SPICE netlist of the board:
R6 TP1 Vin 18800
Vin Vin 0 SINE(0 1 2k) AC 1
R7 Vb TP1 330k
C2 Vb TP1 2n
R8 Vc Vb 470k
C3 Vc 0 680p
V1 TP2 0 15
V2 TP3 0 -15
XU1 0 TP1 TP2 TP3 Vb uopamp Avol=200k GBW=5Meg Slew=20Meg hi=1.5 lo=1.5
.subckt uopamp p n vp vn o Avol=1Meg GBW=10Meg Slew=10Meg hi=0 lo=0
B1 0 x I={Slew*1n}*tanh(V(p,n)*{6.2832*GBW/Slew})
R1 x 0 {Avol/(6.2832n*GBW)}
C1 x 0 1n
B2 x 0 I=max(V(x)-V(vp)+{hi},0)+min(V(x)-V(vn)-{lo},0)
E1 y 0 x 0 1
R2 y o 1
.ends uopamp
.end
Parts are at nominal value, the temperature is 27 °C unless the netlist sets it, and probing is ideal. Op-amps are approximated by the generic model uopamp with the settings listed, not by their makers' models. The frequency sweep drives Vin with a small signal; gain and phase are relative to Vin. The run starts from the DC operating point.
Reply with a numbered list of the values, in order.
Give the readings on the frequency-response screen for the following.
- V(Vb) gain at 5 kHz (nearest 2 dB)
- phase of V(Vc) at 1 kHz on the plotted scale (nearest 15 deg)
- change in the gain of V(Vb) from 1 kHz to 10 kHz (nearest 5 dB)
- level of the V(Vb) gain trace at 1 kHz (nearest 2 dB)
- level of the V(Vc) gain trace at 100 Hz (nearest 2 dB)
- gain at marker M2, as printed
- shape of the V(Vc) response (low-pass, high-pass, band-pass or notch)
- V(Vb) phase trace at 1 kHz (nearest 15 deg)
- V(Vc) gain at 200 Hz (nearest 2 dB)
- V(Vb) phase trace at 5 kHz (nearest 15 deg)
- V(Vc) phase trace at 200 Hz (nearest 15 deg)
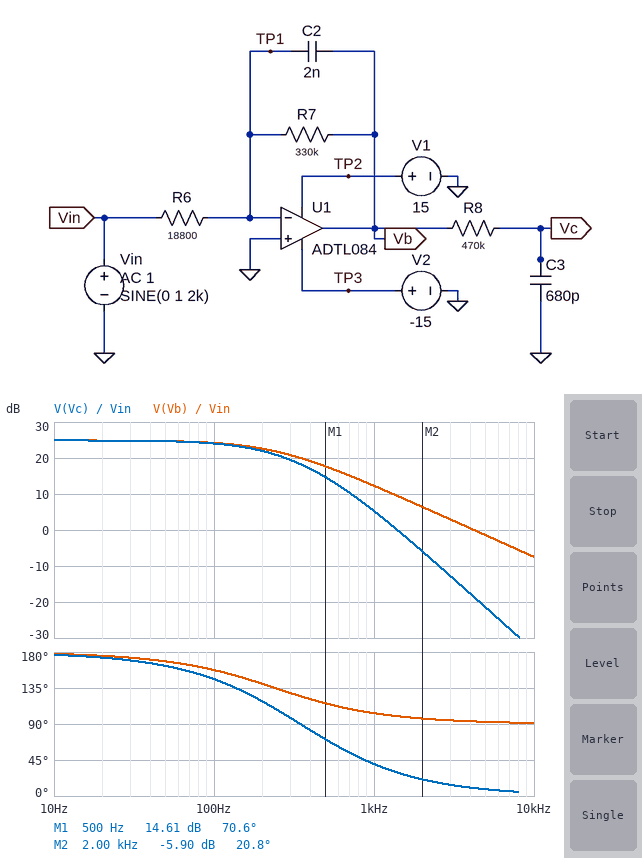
1. -2 dB
2. 45 deg
3. -20 dB
4. 12 dB
5. 24 dB
6. -5.90 dB
7. low-pass
8. 105 deg
9. 22 dB
10. 90 deg
11. 120 deg
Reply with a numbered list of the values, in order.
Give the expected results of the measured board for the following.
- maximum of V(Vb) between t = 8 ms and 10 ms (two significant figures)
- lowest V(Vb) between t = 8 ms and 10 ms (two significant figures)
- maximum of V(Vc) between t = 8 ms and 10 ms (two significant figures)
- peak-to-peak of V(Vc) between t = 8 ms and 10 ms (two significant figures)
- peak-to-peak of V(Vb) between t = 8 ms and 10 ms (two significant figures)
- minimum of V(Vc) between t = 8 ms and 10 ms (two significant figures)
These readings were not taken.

1. 2.1 V
2. -2.1 V
3. 510 mV
4. 1.0 V
5. 4.2 V
6. -510 mV
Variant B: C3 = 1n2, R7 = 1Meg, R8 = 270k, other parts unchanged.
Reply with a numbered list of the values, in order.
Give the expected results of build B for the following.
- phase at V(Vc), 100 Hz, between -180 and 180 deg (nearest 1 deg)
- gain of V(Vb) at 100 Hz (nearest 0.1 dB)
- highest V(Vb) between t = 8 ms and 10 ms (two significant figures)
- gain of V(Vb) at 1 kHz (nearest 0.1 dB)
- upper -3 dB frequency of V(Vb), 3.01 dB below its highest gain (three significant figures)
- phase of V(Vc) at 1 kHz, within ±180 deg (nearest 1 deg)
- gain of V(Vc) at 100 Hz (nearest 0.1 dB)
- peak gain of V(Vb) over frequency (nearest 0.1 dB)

1. 117 deg
2. 30.4 dB
3. 2.1 V
4. 12.5 dB
5. 79.5 Hz
6. 31 deg
7. 30.2 dB
8. 34.5 dB
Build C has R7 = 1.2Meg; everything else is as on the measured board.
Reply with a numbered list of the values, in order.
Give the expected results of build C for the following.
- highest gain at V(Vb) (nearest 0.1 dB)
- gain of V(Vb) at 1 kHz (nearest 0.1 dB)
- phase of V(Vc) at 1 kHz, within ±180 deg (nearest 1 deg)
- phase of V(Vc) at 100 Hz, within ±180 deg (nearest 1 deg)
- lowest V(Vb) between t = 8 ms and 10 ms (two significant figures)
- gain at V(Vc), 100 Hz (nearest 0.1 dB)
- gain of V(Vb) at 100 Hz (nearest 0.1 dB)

1. 36.1 dB
2. 12.5 dB
3. 30 deg
4. 112 deg
5. -2.2 V
6. 30.8 dB
7. 30.9 dB
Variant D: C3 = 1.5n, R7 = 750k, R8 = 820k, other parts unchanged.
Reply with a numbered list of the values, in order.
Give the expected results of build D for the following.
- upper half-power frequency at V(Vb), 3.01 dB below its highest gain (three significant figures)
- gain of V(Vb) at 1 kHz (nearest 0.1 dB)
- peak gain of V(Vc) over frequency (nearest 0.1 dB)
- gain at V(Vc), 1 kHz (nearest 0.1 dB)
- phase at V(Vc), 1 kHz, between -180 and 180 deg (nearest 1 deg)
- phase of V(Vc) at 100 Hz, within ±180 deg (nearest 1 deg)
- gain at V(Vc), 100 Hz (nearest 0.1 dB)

1. 106 Hz
2. 12.5 dB
3. 32.0 dB
4. -5.4 dB
5. 13 deg
6. 99 deg
7. 27.2 dB
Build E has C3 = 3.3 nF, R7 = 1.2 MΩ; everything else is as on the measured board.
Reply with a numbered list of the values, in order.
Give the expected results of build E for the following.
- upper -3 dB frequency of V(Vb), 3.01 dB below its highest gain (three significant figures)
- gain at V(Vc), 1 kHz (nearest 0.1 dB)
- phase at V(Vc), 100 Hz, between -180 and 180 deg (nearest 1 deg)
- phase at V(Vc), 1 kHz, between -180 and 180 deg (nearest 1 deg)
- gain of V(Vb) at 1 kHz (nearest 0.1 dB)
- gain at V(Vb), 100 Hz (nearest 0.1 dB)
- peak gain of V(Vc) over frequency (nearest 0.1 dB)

1. 66.3 Hz
2. -7.3 dB
3. 79 deg
4. 10 deg
5. 12.5 dB
6. 30.9 dB
7. 36.1 dB
